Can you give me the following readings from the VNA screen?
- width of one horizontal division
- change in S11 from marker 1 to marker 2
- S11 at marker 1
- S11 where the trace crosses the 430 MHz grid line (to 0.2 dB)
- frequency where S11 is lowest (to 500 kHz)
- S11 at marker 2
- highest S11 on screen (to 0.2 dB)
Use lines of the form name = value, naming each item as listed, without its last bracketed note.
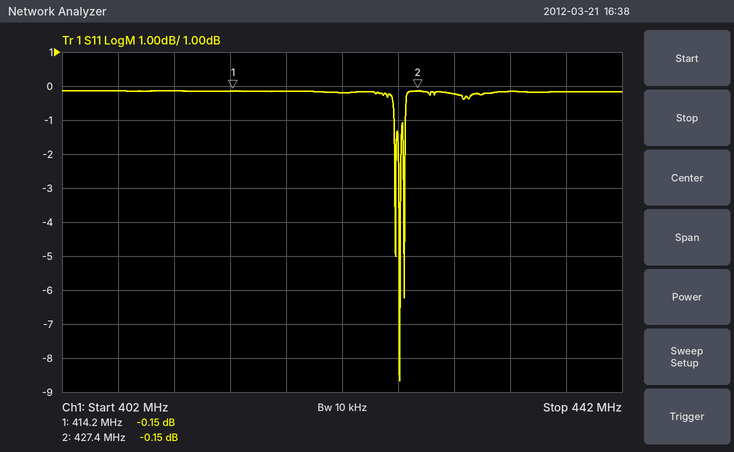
width of one horizontal division = 4 MHz
change in S11 from marker 1 to marker 2 = 0.00 dB
S11 at marker 1 = -0.15 dB
S11 where the trace crosses the 430 MHz grid line = -0.2 dB
frequency where S11 is lowest = 426.0 MHz
S11 at marker 2 = -0.15 dB
highest S11 on screen = -0.2 dB
